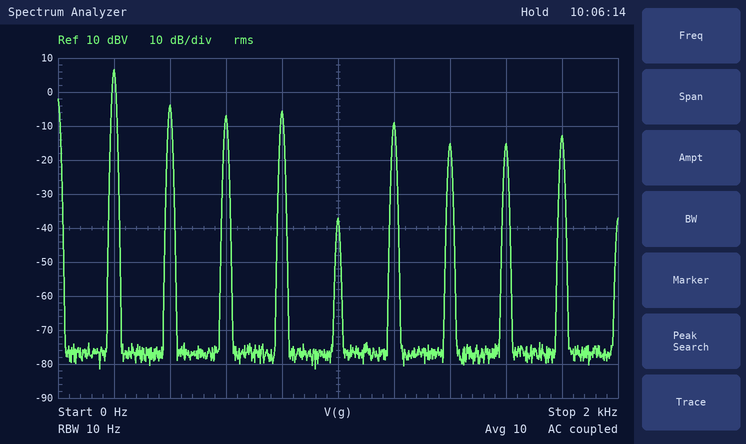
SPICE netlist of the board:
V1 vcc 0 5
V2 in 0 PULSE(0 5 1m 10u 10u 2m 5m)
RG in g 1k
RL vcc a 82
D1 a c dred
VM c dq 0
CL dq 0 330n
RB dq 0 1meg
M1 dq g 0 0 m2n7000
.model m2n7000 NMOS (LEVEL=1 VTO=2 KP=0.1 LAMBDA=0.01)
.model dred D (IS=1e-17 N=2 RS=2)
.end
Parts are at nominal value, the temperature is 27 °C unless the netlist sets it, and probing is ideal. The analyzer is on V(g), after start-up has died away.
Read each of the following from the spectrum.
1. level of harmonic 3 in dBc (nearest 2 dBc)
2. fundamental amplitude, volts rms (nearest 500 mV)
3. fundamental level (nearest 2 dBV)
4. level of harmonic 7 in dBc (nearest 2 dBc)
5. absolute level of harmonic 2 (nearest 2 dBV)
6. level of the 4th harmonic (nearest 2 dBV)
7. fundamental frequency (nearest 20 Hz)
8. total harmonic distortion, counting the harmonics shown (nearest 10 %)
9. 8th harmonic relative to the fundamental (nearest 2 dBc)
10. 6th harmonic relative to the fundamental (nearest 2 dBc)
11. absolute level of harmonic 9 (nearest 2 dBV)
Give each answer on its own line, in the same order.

-14 dBc
2.0 V
6 dBV
-22 dBc
-4 dBV
-6 dBV
200 Hz
50 %
-22 dBc
-16 dBc
-12 dBV
